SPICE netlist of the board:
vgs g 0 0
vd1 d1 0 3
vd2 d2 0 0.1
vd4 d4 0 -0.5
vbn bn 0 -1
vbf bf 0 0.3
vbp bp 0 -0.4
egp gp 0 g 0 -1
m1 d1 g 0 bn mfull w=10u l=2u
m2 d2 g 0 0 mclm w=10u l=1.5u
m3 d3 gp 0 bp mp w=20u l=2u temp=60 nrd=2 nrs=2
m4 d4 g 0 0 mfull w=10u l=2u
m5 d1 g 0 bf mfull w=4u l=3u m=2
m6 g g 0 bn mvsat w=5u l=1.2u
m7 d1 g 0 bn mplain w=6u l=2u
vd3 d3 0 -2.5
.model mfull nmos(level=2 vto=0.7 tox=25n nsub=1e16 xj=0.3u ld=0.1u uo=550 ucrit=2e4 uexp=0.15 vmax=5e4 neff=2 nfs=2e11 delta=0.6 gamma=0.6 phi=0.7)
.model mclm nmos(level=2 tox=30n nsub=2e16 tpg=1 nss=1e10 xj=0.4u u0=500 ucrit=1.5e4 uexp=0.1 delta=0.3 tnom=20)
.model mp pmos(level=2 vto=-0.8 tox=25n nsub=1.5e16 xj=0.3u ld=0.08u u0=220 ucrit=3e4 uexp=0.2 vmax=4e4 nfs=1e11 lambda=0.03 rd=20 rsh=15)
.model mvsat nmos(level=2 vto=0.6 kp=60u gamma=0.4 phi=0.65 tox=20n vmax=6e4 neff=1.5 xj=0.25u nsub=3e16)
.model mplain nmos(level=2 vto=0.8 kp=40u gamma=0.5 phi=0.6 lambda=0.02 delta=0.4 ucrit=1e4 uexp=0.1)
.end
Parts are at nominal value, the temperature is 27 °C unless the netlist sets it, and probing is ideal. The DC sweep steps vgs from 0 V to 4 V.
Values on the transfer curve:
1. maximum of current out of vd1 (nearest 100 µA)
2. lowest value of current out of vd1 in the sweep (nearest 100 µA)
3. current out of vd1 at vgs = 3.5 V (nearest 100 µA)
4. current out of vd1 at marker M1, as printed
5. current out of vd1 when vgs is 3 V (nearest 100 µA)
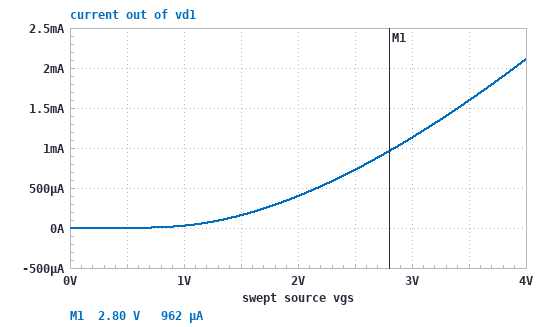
2.1 mA
0 A
1.6 mA
962 µA
1.1 mA
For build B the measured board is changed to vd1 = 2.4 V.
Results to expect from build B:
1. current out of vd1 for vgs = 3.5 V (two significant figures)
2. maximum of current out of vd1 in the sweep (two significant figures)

1.5 mA
2.0 mA
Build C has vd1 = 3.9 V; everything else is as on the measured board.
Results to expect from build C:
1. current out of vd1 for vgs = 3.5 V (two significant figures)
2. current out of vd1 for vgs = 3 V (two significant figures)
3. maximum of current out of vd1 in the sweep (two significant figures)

1.7 mA
1.2 mA
2.2 mA
